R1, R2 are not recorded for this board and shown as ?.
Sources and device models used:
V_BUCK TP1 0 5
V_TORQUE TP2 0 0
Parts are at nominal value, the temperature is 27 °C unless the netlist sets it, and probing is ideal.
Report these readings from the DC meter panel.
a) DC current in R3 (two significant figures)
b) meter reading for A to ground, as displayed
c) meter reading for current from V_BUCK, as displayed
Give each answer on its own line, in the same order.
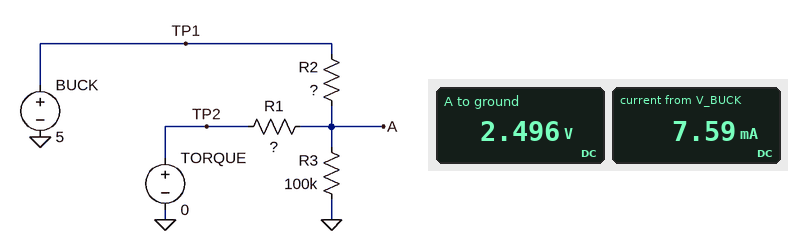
25 µA
2.496 V
7.59 mA
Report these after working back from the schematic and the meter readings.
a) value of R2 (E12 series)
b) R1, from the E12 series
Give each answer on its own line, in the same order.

330 Ω
330 Ω
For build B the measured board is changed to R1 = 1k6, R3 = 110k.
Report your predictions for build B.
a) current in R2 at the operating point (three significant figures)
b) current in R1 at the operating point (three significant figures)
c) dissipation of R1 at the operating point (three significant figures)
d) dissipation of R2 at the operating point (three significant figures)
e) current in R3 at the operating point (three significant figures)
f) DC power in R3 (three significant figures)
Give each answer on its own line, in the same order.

2.62 mA
2.58 mA
10.7 mW
2.27 mW
37.6 µA
155 µW
